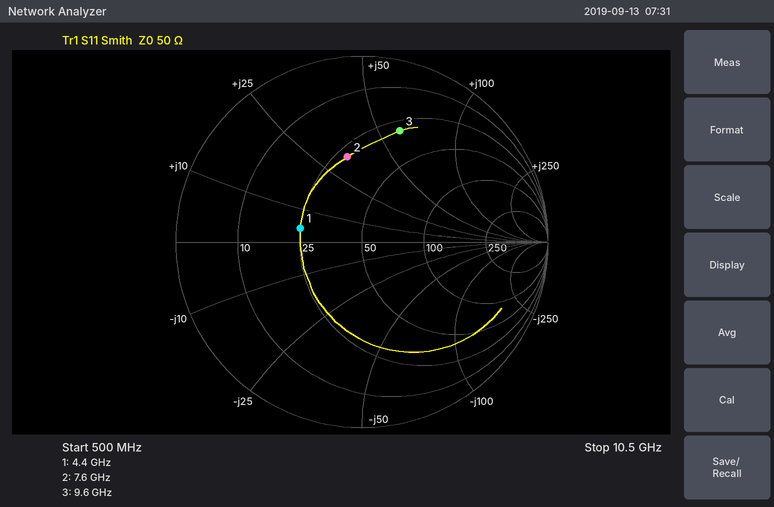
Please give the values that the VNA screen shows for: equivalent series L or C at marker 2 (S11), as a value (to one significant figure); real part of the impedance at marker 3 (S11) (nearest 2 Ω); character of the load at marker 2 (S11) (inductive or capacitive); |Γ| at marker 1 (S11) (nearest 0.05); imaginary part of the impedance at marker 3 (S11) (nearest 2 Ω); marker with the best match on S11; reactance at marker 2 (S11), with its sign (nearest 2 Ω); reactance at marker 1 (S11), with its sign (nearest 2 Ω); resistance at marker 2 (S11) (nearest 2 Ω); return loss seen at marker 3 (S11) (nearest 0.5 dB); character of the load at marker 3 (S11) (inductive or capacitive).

700 pH
30 Ω
inductive
0.35
+60 Ω
marker 1
+34 Ω
+4 Ω
28 Ω
4.0 dB
inductive
